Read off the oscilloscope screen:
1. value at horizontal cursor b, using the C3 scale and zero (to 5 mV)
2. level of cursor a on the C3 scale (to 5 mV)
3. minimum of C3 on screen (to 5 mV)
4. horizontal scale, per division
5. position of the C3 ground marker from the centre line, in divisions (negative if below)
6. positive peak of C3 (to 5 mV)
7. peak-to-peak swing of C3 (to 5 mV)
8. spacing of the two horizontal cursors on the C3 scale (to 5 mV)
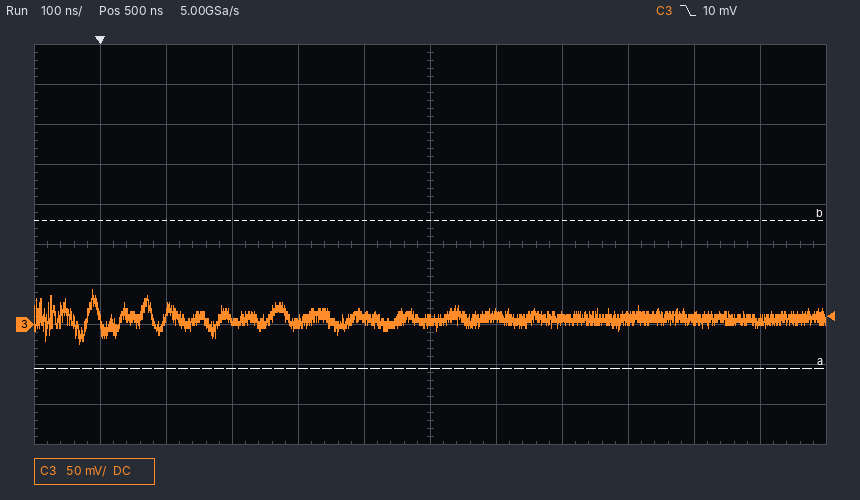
130 mV
-55 mV
-25 mV
100 ns
-2.0 div
45 mV
70 mV
185 mV
